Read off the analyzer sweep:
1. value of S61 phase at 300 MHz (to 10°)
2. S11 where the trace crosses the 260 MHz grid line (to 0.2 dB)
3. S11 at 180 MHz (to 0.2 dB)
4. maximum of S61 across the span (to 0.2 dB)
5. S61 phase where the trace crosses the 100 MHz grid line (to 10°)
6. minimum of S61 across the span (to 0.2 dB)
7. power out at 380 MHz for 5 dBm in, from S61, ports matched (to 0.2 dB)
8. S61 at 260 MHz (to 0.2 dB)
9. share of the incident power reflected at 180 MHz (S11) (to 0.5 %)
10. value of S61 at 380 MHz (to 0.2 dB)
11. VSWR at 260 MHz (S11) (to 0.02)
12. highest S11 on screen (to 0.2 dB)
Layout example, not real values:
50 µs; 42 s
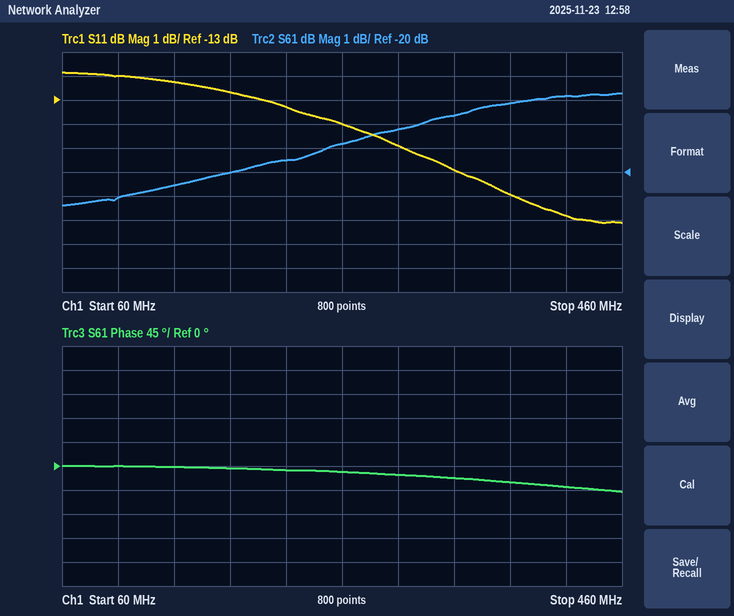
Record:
-20°; -14.0 dB; -12.6 dB; -16.8 dB; 0°; -21.4 dB; -12.2 dBm; -18.8 dB; 5.5 %; -17.2 dB; 1.50; -11.8 dB
